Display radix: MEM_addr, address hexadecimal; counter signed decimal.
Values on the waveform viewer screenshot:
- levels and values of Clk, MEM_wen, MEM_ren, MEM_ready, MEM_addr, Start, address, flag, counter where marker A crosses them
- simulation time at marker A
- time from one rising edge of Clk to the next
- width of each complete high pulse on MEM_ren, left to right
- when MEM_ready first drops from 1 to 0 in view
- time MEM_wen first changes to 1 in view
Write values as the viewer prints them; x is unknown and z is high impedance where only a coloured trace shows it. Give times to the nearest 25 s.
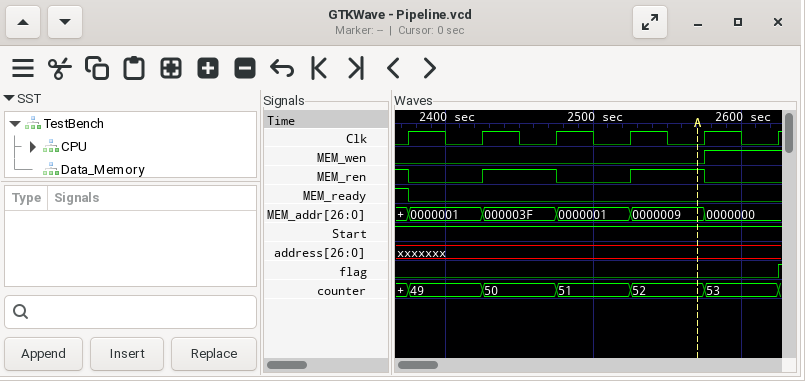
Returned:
Clk=0, MEM_wen=0, MEM_ren=1, MEM_ready=0, MEM_addr=0000009, Start=1, address=xxxxxxx, flag=0, counter=52
2575 s
50 s
50 s, 50 s
2375 s
2575 s
